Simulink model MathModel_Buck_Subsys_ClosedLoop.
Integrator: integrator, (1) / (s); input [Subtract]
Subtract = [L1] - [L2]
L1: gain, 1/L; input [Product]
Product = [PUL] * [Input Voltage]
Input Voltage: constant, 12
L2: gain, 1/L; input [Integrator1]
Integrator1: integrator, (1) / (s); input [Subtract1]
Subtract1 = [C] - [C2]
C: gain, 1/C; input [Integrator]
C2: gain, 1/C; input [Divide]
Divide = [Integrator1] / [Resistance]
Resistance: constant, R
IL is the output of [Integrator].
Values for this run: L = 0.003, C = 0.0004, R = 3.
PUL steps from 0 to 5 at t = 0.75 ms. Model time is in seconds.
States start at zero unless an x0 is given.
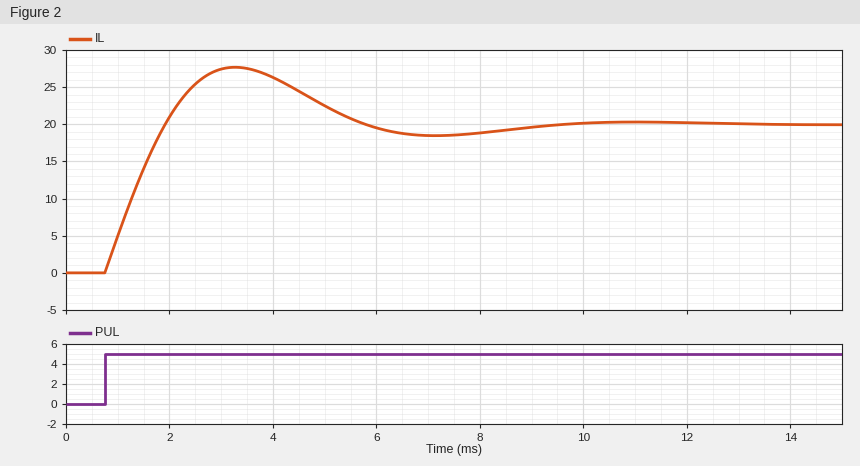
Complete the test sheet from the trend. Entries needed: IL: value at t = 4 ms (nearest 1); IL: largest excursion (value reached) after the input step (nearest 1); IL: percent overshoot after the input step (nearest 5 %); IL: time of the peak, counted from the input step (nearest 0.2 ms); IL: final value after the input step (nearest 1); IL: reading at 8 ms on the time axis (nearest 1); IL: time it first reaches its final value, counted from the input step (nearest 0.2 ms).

26
28
40 %
2.6 ms
20
19
1.2 ms
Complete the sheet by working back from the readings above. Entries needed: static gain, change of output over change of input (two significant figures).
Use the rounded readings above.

4.0
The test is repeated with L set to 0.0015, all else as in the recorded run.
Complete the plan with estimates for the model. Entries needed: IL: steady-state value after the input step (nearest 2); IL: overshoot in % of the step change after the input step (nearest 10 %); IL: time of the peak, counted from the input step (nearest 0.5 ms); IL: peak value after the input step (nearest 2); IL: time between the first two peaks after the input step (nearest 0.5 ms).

20
80 %
1.5 ms
36
5.0 ms
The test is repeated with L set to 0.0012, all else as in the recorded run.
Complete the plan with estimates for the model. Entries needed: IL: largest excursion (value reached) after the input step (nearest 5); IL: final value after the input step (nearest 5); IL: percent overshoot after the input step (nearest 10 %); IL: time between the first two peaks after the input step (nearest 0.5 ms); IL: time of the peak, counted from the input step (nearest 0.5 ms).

40
20
100 %
4.5 ms
1.5 ms
